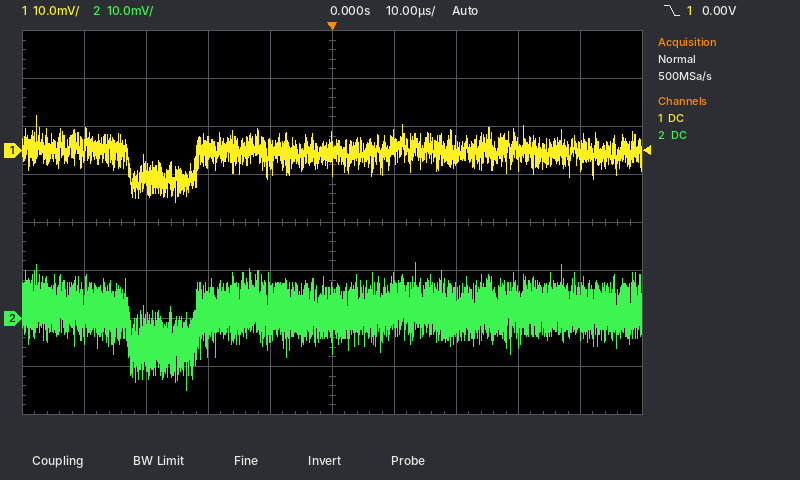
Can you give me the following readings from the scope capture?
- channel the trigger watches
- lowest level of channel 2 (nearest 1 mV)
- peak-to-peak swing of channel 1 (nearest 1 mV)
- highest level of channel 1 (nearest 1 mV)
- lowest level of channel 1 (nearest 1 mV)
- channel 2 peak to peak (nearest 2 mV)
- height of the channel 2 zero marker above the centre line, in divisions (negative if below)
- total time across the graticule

channel 1
-15 mV
18 mV
7 mV
-11 mV
26 mV
-2.0 div
100 µs
